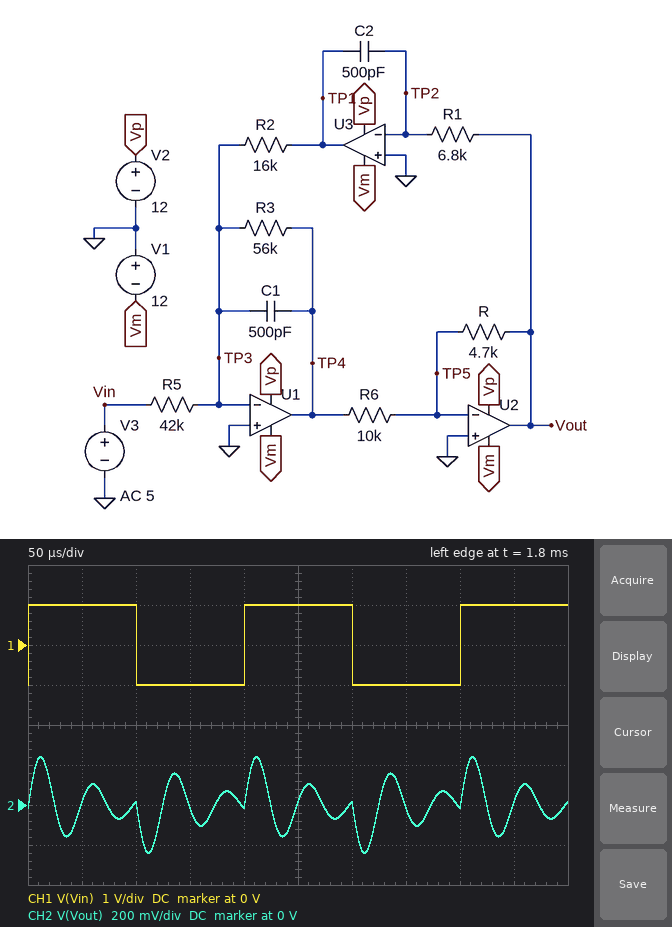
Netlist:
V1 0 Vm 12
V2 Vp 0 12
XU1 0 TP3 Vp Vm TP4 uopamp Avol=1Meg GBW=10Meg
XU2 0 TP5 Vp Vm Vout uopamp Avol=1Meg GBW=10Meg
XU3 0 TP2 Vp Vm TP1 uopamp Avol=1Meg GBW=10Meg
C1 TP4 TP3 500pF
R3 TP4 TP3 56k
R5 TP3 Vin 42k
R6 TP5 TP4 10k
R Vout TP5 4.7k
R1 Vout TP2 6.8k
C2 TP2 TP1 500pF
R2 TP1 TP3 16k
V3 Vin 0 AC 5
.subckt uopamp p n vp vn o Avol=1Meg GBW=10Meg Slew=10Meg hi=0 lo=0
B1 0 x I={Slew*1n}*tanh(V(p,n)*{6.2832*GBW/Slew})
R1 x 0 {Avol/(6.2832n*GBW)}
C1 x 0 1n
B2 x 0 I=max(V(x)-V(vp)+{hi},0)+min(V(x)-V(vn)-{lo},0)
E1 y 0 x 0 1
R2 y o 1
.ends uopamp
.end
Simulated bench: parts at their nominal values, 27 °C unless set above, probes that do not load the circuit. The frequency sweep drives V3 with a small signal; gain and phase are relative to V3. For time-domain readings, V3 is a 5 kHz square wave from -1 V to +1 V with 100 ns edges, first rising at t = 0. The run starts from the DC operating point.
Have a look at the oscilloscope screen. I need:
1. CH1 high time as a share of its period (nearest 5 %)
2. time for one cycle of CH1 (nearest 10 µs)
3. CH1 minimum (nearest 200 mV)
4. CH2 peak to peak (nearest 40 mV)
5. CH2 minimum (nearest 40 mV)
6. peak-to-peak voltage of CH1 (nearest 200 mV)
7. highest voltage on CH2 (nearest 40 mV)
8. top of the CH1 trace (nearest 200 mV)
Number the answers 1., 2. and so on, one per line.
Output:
1. 50 %
2. 200 µs
3. -1.0 V
4. 480 mV
5. -240 mV
6. 2.0 V
7. 240 mV
8. 1.0 V
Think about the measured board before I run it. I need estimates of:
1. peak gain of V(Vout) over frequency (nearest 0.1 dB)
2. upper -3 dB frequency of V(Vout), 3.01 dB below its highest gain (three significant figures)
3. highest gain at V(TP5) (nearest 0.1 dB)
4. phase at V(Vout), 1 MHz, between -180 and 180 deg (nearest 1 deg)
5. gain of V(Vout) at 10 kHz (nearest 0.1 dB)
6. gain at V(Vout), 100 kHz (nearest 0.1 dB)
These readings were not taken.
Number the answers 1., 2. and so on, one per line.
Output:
1. -3.8 dB
2. 23.8 kHz
3. -57.4 dB
4. -104 deg
5. -19.6 dB
6. -28.6 dB
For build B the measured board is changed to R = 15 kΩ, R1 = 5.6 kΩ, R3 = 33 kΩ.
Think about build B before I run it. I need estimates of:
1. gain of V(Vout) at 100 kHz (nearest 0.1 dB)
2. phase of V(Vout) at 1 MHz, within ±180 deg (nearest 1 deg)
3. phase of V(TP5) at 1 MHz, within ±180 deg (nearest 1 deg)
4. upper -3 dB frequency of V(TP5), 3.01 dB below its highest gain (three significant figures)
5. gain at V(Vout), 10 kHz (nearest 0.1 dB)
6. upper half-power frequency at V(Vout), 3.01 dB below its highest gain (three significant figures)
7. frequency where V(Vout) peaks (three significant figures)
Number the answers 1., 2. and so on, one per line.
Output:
1. -17.4 dB
2. -109 deg
3. 161 deg
4. 47.0 kHz
5. -22.9 dB
6. 45.7 kHz
7. 41.0 kHz
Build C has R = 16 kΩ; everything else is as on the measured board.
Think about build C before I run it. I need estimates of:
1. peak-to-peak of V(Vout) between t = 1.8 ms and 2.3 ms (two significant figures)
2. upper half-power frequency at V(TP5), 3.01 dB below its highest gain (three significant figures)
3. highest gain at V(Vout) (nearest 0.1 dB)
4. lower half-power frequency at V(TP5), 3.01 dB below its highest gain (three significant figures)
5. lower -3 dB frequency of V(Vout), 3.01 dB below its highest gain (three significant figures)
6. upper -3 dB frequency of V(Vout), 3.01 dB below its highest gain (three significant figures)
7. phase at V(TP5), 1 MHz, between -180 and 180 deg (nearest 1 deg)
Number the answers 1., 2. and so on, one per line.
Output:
1. 1.0 V
2. 41.4 kHz
3. 7.7 dB
4. 36.3 kHz
5. 36.0 kHz
6. 41.0 kHz
7. 160 deg
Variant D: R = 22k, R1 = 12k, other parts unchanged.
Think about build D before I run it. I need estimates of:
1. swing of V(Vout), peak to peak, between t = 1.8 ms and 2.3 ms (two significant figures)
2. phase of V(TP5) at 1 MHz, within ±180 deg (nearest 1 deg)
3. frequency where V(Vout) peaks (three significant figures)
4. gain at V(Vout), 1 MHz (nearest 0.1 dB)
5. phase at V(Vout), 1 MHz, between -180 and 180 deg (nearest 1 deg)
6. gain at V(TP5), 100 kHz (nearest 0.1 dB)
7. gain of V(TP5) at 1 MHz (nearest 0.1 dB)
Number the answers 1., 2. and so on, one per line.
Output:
1. 2.0 V
2. 157 deg
3. 34.0 kHz
4. -36.0 dB
5. -113 deg
6. -54.5 dB
7. -56.0 dB
